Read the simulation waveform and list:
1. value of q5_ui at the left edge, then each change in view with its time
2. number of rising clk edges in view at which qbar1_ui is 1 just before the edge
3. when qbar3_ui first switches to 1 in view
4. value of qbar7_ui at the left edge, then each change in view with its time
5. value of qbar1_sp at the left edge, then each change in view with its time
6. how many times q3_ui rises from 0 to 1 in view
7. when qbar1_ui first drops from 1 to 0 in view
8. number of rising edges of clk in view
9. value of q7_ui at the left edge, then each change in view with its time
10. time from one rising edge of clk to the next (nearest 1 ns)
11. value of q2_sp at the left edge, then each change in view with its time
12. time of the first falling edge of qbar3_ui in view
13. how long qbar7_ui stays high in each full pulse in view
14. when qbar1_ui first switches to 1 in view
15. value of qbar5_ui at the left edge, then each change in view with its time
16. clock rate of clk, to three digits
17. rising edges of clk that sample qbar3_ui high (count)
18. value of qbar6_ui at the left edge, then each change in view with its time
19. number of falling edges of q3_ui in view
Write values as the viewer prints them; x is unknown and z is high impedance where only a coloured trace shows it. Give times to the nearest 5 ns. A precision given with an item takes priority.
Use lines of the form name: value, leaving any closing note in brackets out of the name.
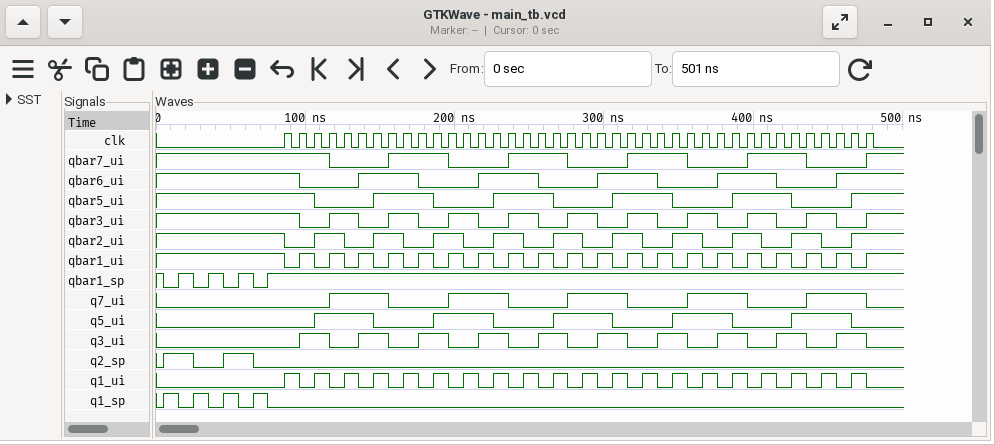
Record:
value of q5_ui at the left edge, then each change in view with its time: 0, 1 at 105 ns, 0 at 145 ns, 1 at 185 ns, 0 at 225 ns, 1 at 265 ns, 0 at 305 ns, 1 at 345 ns, 0 at 385 ns, 1 at 425 ns, 0 at 465 ns
number of rising clk edges in view at which qbar1_ui is 1 just before the edge: 20
when qbar3_ui first switches to 1 in view: 115 ns
value of qbar7_ui at the left edge, then each change in view with its time: 1, 0 at 115 ns, 1 at 155 ns, 0 at 195 ns, 1 at 235 ns, 0 at 275 ns, 1 at 315 ns, 0 at 355 ns, 1 at 395 ns, 0 at 435 ns, 1 at 475 ns
value of qbar1_sp at the left edge, then each change in view with its time: 1, 0 at 5 ns, 1 at 15 ns, 0 at 25 ns, 1 at 35 ns, 0 at 45 ns, 1 at 55 ns, 0 at 65 ns, 1 at 75 ns
how many times q3_ui rises from 0 to 1 in view: 10
when qbar1_ui first drops from 1 to 0 in view: 85 ns
number of rising edges of clk in view: 40
value of q7_ui at the left edge, then each change in view with its time: 0, 1 at 115 ns, 0 at 155 ns, 1 at 195 ns, 0 at 235 ns, 1 at 275 ns, 0 at 315 ns, 1 at 355 ns, 0 at 395 ns, 1 at 435 ns, 0 at 475 ns
time from one rising edge of clk to the next: 10 ns
value of q2_sp at the left edge, then each change in view with its time: 0, 1 at 5 ns, 0 at 25 ns, 1 at 45 ns, 0 at 65 ns
time of the first falling edge of qbar3_ui in view: 95 ns
how long qbar7_ui stays high in each full pulse in view: 40 ns, 40 ns, 40 ns, 40 ns
when qbar1_ui first switches to 1 in view: 95 ns
value of qbar5_ui at the left edge, then each change in view with its time: 1, 0 at 105 ns, 1 at 145 ns, 0 at 185 ns, 1 at 225 ns, 0 at 265 ns, 1 at 305 ns, 0 at 345 ns, 1 at 385 ns, 0 at 425 ns, 1 at 465 ns
clock rate of clk, to three digits: 100 MHz
rising edges of clk that sample qbar3_ui high: 20
value of qbar6_ui at the left edge, then each change in view with its time: 1, 0 at 95 ns, 1 at 135 ns, 0 at 175 ns, 1 at 215 ns, 0 at 255 ns, 1 at 295 ns, 0 at 335 ns, 1 at 375 ns, 0 at 415 ns, 1 at 455 ns
number of falling edges of q3_ui in view: 10
